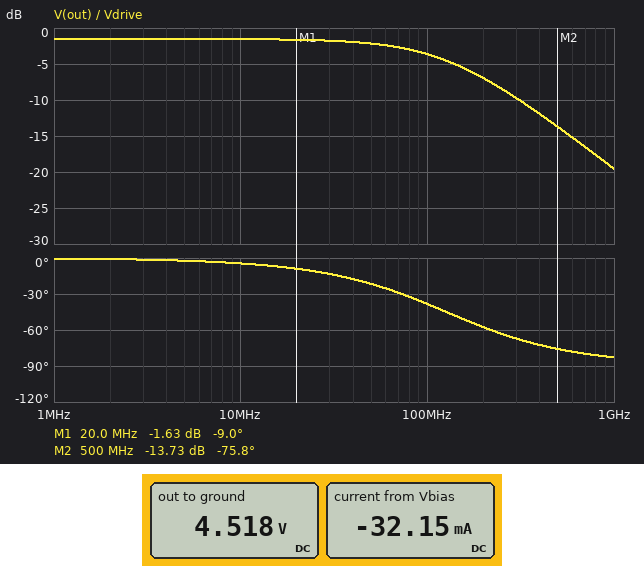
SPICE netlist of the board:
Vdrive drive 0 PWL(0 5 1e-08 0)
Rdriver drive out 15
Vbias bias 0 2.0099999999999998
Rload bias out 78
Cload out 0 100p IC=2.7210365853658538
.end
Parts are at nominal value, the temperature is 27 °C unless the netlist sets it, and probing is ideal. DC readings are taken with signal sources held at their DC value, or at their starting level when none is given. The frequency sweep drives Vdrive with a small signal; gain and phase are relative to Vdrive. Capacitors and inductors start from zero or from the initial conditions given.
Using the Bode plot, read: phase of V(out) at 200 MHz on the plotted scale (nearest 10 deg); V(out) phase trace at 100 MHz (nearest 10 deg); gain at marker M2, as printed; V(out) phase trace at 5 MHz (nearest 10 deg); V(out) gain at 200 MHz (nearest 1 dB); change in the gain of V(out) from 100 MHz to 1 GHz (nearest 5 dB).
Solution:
-60 deg
-40 deg
-13.73 dB
0 deg
-7 dB
-15 dB
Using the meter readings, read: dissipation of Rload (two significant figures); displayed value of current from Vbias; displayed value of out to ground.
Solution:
81 mW
-32.15 mA
4.518 V
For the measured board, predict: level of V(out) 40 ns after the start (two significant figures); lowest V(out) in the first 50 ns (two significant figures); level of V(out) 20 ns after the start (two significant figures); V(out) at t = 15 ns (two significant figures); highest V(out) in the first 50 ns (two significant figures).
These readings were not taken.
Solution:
320 mV
320 mV
320 mV
330 mV
3.7 V
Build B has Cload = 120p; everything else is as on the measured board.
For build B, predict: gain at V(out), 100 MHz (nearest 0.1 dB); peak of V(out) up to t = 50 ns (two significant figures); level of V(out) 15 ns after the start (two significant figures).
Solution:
-4.3 dB
3.7 V
350 mV
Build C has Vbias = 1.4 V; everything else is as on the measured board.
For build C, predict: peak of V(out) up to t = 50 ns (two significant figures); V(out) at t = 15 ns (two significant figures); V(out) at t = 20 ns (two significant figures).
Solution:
3.7 V
240 mV
230 mV
